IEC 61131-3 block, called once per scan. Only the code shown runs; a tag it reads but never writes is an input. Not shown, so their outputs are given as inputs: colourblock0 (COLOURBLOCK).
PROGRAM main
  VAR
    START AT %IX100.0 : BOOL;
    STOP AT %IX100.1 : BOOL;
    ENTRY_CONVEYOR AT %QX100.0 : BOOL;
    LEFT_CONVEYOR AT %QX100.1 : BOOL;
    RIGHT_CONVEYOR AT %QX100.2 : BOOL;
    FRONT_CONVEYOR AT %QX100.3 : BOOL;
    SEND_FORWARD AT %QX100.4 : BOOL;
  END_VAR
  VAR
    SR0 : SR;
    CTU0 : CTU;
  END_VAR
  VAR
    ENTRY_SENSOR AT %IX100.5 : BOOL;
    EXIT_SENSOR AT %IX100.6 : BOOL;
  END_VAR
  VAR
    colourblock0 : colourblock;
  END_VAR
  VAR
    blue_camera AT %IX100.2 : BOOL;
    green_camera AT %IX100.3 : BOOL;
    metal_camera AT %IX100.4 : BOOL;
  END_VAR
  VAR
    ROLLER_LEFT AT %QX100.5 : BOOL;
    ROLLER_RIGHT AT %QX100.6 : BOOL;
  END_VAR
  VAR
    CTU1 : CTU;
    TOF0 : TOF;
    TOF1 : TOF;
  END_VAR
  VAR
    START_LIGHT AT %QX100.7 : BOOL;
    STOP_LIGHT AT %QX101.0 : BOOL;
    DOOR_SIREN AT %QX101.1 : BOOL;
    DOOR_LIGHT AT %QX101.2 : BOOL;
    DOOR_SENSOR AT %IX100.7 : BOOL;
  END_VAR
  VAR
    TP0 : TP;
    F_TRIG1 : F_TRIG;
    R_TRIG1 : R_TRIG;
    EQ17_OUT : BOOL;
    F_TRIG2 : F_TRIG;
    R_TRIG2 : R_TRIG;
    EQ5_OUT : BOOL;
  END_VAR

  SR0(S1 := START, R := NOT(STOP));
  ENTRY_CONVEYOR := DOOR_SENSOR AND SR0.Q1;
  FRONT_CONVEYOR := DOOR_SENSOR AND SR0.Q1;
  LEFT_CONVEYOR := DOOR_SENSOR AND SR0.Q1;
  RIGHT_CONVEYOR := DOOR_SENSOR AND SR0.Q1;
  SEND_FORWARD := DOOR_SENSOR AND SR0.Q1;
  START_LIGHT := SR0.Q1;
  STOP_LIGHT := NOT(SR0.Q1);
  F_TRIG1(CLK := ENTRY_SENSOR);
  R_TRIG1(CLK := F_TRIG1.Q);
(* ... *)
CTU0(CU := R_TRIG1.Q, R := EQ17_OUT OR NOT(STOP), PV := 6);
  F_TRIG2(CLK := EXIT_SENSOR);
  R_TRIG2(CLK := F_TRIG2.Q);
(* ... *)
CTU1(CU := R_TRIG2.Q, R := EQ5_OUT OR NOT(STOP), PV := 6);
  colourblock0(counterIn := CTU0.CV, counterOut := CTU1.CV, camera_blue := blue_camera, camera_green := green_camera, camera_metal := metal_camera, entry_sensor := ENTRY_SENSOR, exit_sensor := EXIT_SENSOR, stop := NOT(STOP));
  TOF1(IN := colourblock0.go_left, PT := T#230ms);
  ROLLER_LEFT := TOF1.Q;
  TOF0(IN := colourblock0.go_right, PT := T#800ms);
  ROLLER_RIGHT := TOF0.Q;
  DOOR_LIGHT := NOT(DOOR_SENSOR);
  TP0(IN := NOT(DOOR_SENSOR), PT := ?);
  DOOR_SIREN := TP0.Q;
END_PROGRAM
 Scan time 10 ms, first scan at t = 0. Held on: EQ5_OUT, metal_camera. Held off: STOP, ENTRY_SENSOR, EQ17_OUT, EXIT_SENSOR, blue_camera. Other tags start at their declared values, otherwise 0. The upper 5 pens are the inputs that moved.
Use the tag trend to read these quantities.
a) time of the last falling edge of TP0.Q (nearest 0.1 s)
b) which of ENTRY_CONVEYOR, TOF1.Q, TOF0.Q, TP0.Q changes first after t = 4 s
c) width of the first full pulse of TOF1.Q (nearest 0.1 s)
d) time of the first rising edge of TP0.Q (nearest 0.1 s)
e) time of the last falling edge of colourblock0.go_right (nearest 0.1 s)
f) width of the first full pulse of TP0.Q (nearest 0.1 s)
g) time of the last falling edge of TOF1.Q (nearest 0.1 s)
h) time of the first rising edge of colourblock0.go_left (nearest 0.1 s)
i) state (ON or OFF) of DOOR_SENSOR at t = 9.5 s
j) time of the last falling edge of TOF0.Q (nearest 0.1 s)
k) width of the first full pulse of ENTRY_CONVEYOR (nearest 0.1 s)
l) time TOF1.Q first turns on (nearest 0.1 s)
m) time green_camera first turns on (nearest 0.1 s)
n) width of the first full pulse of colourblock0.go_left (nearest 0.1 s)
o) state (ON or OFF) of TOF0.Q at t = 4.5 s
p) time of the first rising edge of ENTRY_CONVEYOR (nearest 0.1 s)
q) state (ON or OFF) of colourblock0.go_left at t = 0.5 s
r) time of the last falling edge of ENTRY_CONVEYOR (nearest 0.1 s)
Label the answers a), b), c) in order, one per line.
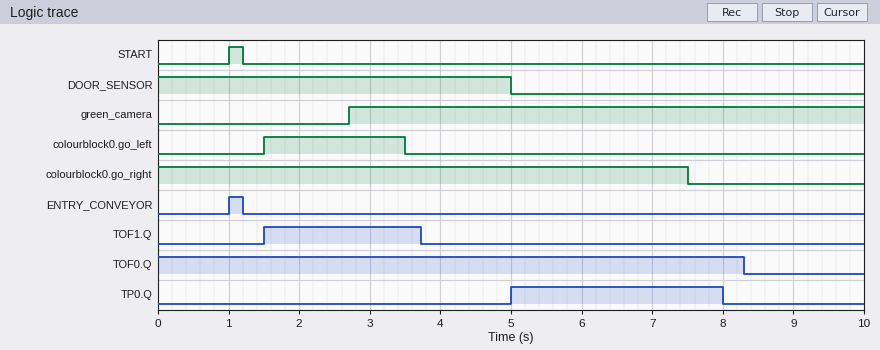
a) 8.0 s
b) TP0.Q
c) 2.2 s
d) 5.0 s
e) 7.5 s
f) 3.0 s
g) 3.7 s
h) 1.5 s
i) OFF
j) 8.3 s
k) 0.2 s
l) 1.5 s
m) 2.7 s
n) 2.0 s
o) ON
p) 1.0 s
q) OFF
r) 1.2 s
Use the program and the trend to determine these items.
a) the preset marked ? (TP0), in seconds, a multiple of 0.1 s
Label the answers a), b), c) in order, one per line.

a) 3.0 s
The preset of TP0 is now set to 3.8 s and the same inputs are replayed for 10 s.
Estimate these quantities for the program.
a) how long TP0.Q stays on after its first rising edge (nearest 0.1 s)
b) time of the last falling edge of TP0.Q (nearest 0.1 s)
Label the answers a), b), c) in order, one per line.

a) 3.8 s
b) 8.8 s
